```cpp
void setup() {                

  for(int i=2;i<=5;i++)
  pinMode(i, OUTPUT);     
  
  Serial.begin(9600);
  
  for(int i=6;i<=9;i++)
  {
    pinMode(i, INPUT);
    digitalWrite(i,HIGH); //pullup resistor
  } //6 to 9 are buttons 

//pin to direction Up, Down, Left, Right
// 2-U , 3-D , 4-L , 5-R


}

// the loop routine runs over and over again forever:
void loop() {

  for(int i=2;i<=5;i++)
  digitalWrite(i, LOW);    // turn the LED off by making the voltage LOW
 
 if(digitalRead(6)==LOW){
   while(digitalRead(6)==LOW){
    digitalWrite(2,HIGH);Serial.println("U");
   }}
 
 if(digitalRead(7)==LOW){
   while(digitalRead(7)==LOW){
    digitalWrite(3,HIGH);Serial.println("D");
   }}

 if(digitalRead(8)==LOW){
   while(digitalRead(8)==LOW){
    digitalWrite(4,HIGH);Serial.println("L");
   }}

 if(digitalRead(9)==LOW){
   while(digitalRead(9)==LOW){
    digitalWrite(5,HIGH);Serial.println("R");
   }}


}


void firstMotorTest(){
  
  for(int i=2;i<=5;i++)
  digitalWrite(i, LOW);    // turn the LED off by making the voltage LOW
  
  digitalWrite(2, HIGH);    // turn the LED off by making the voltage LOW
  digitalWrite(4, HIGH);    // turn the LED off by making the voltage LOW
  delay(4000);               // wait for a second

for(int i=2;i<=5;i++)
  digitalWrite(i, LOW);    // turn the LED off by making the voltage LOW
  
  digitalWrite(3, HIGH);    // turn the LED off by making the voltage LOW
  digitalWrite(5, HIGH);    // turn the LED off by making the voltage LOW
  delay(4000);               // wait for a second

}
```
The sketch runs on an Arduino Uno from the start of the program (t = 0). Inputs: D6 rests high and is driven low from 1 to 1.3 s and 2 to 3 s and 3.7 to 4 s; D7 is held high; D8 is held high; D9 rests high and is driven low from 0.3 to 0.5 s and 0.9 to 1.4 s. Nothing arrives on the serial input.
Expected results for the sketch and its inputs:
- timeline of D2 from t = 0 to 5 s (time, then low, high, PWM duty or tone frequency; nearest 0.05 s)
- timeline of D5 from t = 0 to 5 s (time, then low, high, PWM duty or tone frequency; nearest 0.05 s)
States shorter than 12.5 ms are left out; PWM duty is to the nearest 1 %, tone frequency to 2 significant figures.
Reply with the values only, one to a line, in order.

0 s low; 2 s high; 3 s low; 3.7 s high; 4 s low
0 s low; 0.3 s high; 0.5 s low; 0.9 s high; 1.4 s low
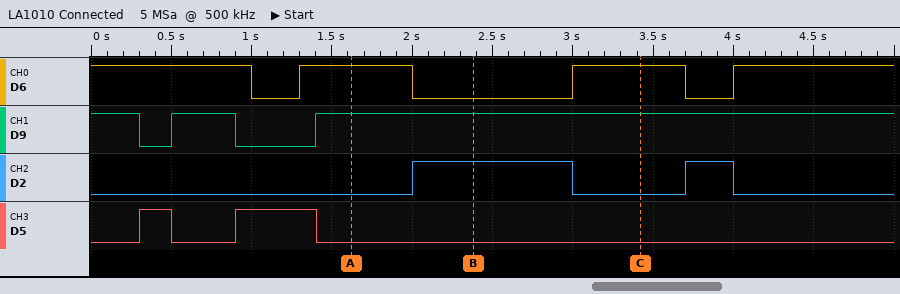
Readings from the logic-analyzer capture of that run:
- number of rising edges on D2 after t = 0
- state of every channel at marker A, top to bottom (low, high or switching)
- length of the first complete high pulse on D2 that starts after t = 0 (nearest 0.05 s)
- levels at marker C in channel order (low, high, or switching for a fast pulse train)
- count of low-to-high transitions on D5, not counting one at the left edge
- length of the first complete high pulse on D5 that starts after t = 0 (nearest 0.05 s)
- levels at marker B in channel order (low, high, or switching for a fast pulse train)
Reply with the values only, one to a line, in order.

2
D6 high, D9 high, D2 low, D5 low
1.00 s
D6 high, D9 high, D2 low, D5 low
2
0.20 s
D6 low, D9 high, D2 high, D5 low
